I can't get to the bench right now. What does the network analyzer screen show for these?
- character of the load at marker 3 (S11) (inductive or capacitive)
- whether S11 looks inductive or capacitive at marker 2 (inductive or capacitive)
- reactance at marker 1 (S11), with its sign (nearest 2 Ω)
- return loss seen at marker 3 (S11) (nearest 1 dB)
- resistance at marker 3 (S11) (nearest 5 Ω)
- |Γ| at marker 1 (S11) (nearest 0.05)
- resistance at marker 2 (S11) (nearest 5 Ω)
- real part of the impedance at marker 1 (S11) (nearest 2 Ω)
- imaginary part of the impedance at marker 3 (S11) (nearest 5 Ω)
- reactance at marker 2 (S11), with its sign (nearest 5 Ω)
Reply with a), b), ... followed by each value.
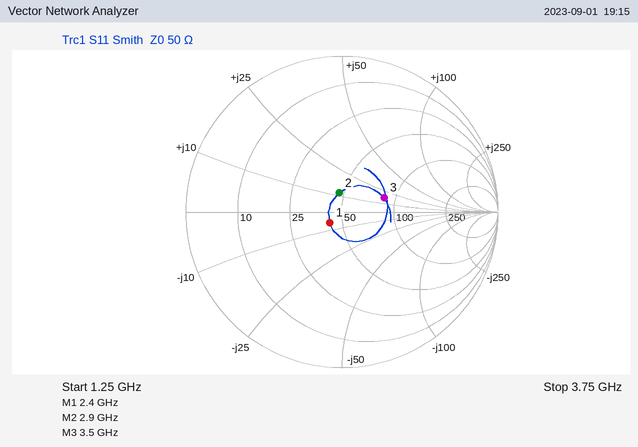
a) inductive
b) inductive
c) -6 Ω
d) 11 dB
e) 85 Ω
f) 0.10
g) 45 Ω
h) 42 Ω
i) +15 Ω
j) +10 Ω
